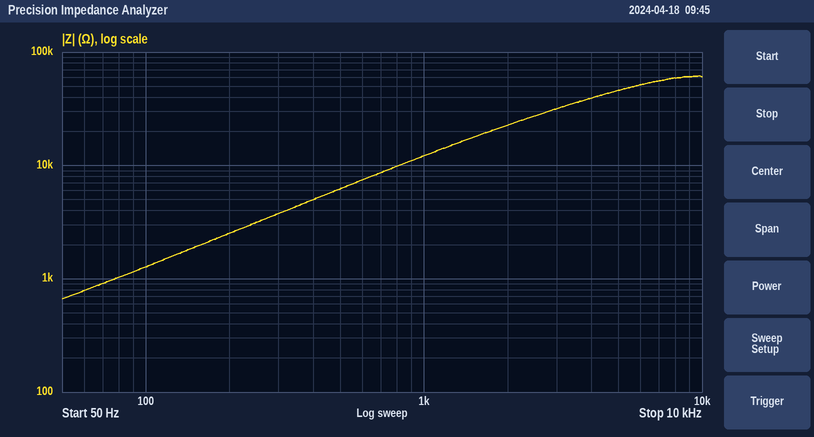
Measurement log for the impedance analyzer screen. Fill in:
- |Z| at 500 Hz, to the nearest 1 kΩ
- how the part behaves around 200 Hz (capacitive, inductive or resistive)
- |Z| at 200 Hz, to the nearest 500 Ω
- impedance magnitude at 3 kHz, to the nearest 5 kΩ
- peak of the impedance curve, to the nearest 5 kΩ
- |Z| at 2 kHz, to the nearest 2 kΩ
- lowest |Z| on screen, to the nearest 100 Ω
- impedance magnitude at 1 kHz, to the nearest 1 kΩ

6 kΩ
inductive
2.5 kΩ
30 kΩ
60 kΩ
22 kΩ
700 Ω
12 kΩ
